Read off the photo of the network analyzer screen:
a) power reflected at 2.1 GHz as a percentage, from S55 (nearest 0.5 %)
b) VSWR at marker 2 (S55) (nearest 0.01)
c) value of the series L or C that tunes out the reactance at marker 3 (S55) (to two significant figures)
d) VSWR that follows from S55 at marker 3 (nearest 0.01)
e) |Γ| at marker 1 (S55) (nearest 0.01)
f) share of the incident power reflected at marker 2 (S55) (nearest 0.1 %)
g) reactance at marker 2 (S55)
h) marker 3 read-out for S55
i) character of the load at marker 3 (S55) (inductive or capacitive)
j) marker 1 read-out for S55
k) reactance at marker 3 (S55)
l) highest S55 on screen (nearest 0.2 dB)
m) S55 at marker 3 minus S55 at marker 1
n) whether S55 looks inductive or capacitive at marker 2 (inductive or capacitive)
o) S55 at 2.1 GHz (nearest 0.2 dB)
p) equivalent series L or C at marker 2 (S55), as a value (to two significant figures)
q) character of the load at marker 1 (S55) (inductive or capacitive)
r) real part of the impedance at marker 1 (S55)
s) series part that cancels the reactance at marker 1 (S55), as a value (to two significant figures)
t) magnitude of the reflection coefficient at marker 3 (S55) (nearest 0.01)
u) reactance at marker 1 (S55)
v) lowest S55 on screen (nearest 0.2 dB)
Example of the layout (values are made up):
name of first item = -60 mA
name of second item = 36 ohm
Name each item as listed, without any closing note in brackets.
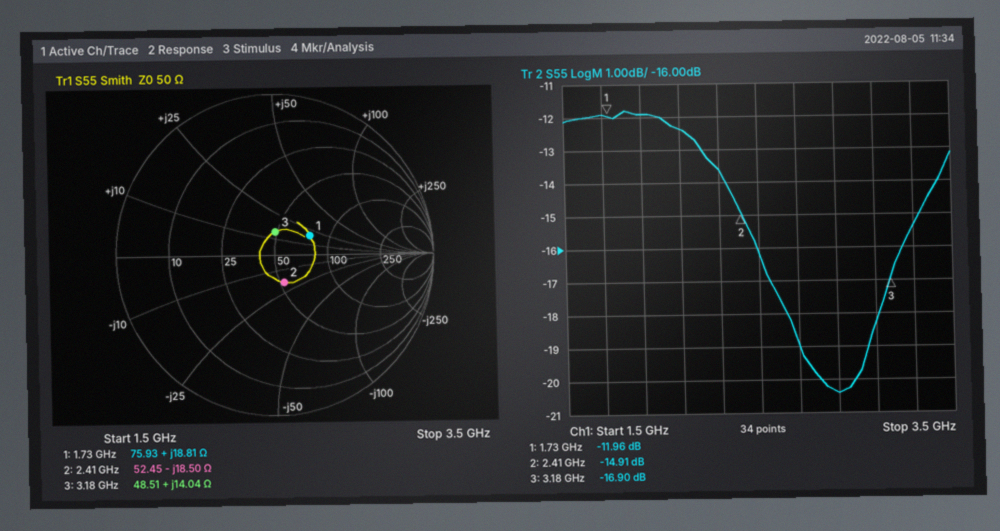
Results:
power reflected at 2.1 GHz as a percentage, from S55 = 6.0 %
VSWR at marker 2 (S55) = 1.44
value of the series L or C that tunes out the reactance at marker 3 (S55) = 3.6 pF
VSWR that follows from S55 at marker 3 = 1.33
|Γ| at marker 1 (S55) = 0.25
share of the incident power reflected at marker 2 (S55) = 3.2 %
reactance at marker 2 = -18.50 Ω
marker 3 read-out for S55 = -16.90 dB
character of the load at marker 3 (S55) = inductive
marker 1 read-out for S55 = -11.96 dB
reactance at marker 3 = +14.04 Ω
highest S55 on screen = -11.8 dB
S55 at marker 3 minus S55 at marker 1 = -4.94 dB
whether S55 looks inductive or capacitive at marker 2 = capacitive
S55 at 2.1 GHz = -12.4 dB
equivalent series L or C at marker 2 (S55), as a value = 3.6 pF
character of the load at marker 1 (S55) = inductive
real part of the impedance at marker 1 = 75.93 Ω
series part that cancels the reactance at marker 1 (S55), as a value = 4.9 pF
magnitude of the reflection coefficient at marker 3 (S55) = 0.14
reactance at marker 1 = +18.81 Ω
lowest S55 on screen = -20.4 dB
